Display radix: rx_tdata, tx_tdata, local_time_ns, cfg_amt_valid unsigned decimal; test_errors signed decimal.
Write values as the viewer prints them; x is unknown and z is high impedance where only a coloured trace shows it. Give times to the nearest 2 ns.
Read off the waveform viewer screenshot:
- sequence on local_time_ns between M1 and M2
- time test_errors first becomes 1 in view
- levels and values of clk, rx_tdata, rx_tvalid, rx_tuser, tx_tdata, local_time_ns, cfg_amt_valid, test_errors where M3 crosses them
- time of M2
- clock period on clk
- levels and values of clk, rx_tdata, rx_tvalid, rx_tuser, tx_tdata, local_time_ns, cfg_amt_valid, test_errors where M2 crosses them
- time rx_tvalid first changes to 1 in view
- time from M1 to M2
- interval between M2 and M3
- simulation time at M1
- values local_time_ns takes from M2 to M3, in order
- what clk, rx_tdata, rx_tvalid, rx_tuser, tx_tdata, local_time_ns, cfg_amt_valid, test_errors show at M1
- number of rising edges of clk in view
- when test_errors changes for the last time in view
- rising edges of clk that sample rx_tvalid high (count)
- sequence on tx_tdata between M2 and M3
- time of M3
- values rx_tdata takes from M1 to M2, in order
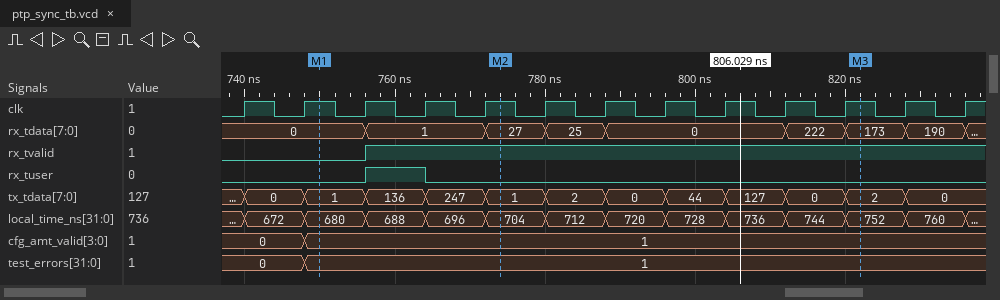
680, 688, 696, 704
748 ns
clk=1, rx_tdata=173, rx_tvalid=1, rx_tuser=0, tx_tdata=2, local_time_ns=752, cfg_amt_valid=1, test_errors=1
774 ns
8 ns
clk=1, rx_tdata=27, rx_tvalid=1, rx_tuser=0, tx_tdata=1, local_time_ns=704, cfg_amt_valid=1, test_errors=1
756 ns
24 ns
48 ns
750 ns
704, 712, 720, 728, 736, 744, 752
clk=1, rx_tdata=0, rx_tvalid=0, rx_tuser=0, tx_tdata=1, local_time_ns=680, cfg_amt_valid=1, test_errors=1
13
748 ns
10
1, 2, 0, 44, 127, 0, 2
822 ns
0, 1, 27
